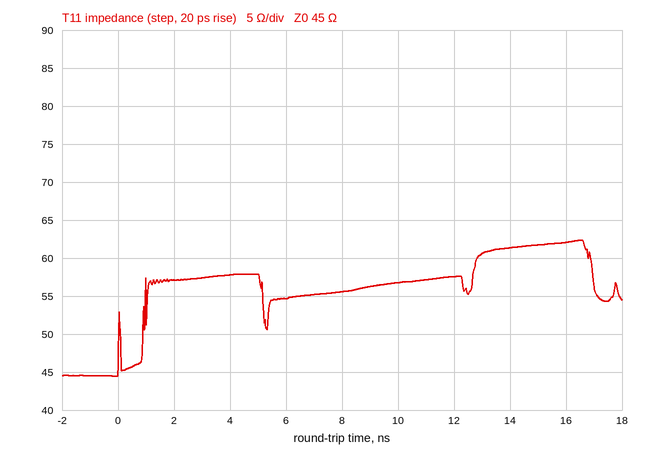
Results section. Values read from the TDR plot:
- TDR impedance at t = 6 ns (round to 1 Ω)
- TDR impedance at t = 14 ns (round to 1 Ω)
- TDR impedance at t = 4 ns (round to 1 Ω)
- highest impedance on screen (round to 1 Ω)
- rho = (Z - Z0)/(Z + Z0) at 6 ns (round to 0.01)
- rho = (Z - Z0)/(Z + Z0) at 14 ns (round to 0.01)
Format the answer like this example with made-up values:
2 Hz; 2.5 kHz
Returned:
55 Ω; 61 Ω; 58 Ω; 62 Ω; +0.10; +0.15
